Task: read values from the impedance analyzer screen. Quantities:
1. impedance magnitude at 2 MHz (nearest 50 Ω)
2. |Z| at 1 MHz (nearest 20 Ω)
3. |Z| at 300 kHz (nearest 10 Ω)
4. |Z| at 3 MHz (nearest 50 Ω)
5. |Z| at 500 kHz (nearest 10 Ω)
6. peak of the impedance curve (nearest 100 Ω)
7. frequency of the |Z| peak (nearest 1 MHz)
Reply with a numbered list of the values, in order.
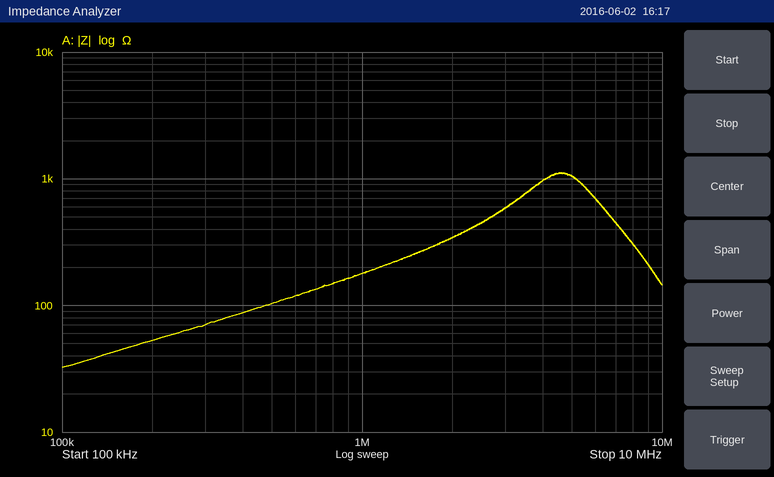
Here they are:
1. 350 Ω
2. 180 Ω
3. 70 Ω
4. 600 Ω
5. 100 Ω
6. 1.1 kΩ
7. 5 MHz
